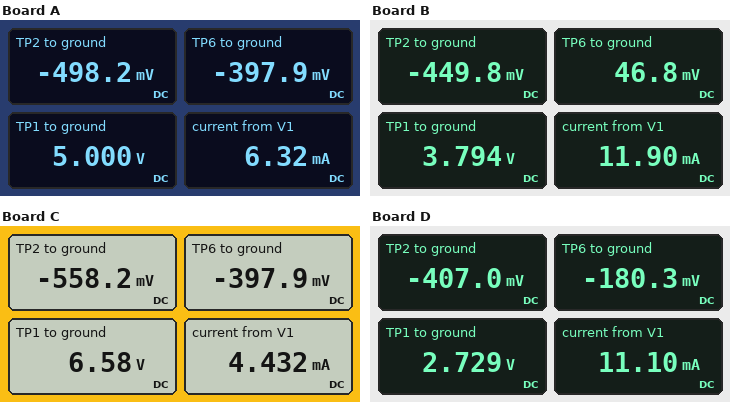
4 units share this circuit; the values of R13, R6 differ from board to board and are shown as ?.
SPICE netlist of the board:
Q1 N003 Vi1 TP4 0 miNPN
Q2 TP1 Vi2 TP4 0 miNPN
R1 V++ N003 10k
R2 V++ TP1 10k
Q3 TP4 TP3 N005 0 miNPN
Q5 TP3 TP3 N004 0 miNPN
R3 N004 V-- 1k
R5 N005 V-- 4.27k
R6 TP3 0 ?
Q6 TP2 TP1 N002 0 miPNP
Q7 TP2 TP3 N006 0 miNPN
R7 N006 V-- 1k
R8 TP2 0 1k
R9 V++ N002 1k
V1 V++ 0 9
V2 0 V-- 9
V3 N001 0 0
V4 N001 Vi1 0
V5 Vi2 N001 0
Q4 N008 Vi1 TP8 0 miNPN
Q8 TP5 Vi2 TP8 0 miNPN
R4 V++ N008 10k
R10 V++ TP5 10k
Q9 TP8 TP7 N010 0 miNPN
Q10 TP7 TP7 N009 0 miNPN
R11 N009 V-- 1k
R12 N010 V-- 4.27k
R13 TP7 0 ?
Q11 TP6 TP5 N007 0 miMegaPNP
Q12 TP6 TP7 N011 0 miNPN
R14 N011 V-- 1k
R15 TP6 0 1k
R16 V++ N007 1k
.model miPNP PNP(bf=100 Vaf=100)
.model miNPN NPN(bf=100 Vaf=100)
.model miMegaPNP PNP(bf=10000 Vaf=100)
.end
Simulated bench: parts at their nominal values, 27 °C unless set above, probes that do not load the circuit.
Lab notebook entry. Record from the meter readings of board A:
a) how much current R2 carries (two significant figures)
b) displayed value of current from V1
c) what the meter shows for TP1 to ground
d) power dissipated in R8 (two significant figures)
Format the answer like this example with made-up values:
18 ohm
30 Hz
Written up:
400 µA
6.32 mA
5.000 V
250 µW
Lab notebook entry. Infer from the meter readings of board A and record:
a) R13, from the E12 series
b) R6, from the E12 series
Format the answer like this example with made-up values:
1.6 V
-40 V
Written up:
2.7 kΩ
1.2 kΩ
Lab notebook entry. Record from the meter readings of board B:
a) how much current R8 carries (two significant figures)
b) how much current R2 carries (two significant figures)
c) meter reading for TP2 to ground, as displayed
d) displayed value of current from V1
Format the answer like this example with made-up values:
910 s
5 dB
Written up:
450 µA
520 µA
-449.8 mV
11.90 mA
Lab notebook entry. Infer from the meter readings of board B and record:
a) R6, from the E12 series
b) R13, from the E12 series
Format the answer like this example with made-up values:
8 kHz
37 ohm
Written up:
680 Ω
560 Ω
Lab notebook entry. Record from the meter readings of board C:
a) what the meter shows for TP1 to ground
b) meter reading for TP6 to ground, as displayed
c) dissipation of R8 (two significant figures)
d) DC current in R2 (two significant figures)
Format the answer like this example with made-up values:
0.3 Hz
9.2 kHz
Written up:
6.58 V
-397.9 mV
310 µW
240 µA
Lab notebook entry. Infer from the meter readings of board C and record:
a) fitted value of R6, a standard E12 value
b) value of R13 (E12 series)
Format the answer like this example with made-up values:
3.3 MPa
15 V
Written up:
2.7 kΩ
2.7 kΩ
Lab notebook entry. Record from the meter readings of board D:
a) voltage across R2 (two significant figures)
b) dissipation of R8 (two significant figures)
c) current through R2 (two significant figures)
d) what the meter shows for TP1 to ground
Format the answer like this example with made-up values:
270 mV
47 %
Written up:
6.3 V
170 µW
630 µA
2.729 V
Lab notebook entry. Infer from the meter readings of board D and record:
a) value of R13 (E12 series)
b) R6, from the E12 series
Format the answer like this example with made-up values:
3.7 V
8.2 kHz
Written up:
1.2 kΩ
390 Ω
